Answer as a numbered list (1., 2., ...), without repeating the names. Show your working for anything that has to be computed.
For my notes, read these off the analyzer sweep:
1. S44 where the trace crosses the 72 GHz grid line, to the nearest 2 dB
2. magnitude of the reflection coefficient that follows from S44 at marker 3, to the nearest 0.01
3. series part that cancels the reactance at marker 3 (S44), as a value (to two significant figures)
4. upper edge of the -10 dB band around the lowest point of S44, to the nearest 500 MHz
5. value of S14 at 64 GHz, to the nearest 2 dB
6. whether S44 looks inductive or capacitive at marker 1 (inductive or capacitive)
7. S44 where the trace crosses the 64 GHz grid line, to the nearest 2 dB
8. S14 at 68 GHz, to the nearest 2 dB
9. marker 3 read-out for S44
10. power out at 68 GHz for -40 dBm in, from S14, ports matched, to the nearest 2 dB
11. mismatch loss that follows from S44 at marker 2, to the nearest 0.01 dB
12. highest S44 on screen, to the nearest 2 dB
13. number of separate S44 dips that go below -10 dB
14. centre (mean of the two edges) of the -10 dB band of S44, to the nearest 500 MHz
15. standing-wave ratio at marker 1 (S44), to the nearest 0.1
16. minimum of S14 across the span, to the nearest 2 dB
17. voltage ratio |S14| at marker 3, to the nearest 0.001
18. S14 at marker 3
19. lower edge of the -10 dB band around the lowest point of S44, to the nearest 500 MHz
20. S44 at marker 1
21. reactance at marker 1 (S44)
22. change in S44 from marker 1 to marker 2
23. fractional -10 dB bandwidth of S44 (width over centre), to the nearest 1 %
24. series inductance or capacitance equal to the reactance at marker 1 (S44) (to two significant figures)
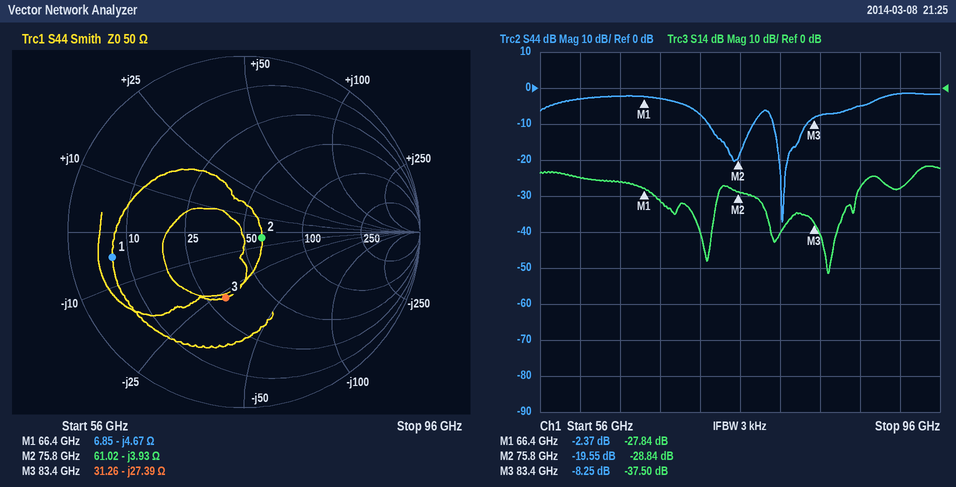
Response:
1. -8 dB
2. 10^(-8.25/20) ≈ 0.39
3. L = 27.39 Ω/(2π × 83.4 GHz) ≈ 52 pH
4. 82.5 GHz
5. -26 dB
6. capacitive
7. -2 dB
8. -32 dB
9. -8.25 dB
10. -40 dBm + (-32 dB) = -72 dBm
11. −10 log10(1 − 10^(-19.55/10)) ≈ 0.05 dB
12. -2 dB
13. 2
14. 81.0 GHz
15. 7.4
16. -52 dB
17. 10^(-37.5/20) ≈ 0.013
18. -37.50 dB
19. 79.5 GHz
20. -2.37 dB
21. -4.67 Ω
22. -19.55 − (-2.37) = -17.18 dB
23. 3 GHz / 81 GHz ≈ 4 %
24. C = 1/(2π × 66.4 GHz × 4.67 Ω) ≈ 513 fF, so 510 fF to two significant figures
